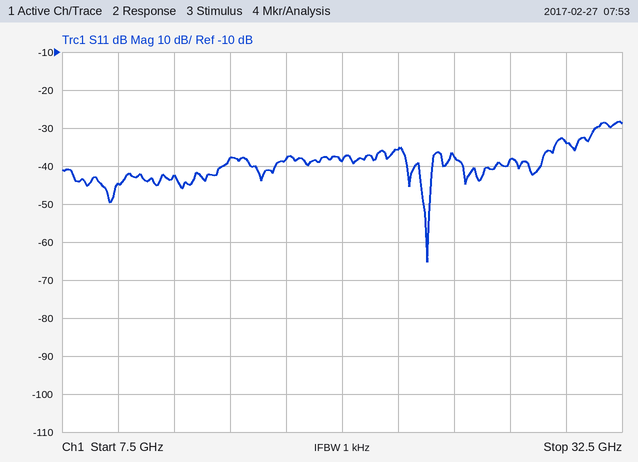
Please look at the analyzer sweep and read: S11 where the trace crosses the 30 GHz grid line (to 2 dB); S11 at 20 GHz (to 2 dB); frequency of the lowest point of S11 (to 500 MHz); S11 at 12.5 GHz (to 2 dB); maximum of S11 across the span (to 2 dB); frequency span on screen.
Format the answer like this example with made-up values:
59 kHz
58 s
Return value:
-34 dB
-38 dB
24.0 GHz
-42 dB
-28 dB
25 GHz
